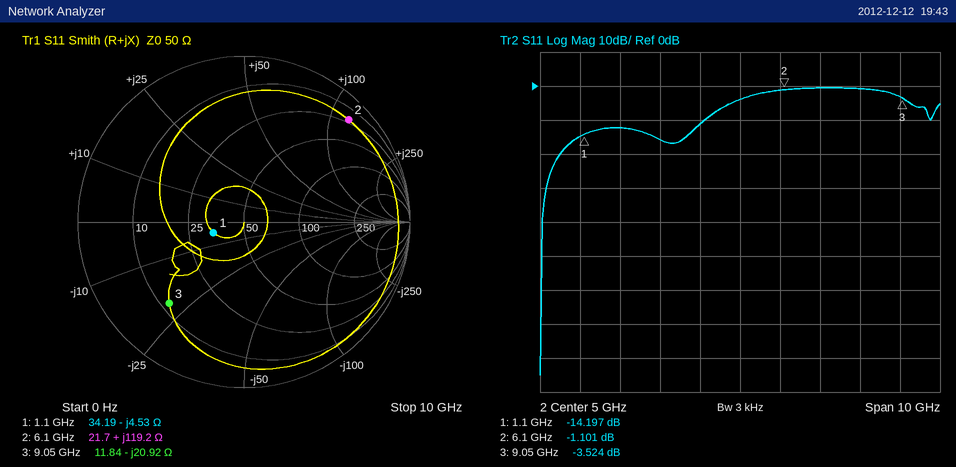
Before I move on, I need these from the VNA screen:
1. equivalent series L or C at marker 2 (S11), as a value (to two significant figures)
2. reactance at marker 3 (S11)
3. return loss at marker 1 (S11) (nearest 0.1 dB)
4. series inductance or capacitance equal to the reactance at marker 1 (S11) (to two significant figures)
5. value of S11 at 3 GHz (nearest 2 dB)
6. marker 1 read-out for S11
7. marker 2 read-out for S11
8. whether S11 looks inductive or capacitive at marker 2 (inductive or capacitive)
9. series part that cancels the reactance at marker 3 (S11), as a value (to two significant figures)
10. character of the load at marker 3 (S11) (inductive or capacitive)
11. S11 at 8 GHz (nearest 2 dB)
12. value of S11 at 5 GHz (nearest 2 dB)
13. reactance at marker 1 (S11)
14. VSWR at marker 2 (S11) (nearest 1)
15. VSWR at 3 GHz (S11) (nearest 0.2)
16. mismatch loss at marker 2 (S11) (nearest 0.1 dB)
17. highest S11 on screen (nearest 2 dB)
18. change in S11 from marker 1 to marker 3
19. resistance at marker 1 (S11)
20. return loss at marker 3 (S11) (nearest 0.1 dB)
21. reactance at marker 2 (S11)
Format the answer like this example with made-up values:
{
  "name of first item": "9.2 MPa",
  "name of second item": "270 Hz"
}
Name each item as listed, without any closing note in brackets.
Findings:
{
  "equivalent series L or C at marker 2 (S11), as a value": "3.1 nH",
  "reactance at marker 3": "-20.92 Ω",
  "return loss at marker 1 (S11)": "14.2 dB",
  "series inductance or capacitance equal to the reactance at marker 1 (S11)": "32 pF",
  "value of S11 at 3 GHz": "-16 dB",
  "marker 1 read-out for S11": "-14.197 dB",
  "marker 2 read-out for S11": "-1.101 dB",
  "whether S11 looks inductive or capacitive at marker 2": "inductive",
  "series part that cancels the reactance at marker 3 (S11), as a value": "370 pH",
  "character of the load at marker 3 (S11)": "capacitive",
  "S11 at 8 GHz": "0 dB",
  "value of S11 at 5 GHz": "-4 dB",
  "reactance at marker 1": "-4.53 Ω",
  "VSWR at marker 2 (S11)": "16",
  "VSWR at 3 GHz (S11)": "1.4",
  "mismatch loss at marker 2 (S11)": "6.5 dB",
  "highest S11 on screen": "0 dB",
  "change in S11 from marker 1 to marker 3": "10.673 dB",
  "resistance at marker 1": "34.19 Ω",
  "return loss at marker 3 (S11)": "3.5 dB",
  "reactance at marker 2": "+119.2 Ω"
}
